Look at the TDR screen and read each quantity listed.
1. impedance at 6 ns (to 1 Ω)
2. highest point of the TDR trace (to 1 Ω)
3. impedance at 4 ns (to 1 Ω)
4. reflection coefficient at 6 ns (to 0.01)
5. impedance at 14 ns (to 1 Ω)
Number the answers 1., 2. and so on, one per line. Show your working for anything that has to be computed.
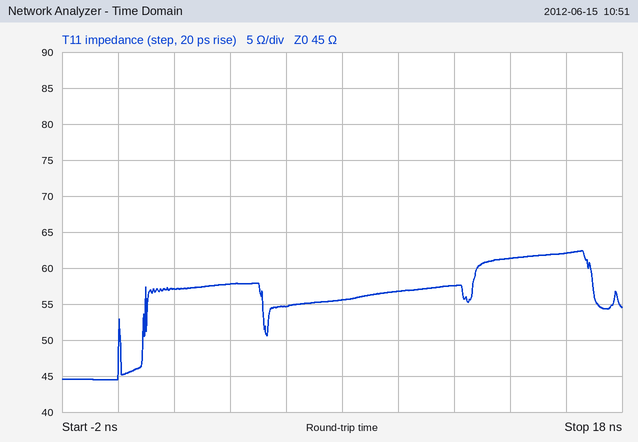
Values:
1. 55 Ω
2. 62 Ω
3. 58 Ω
4. (55 − 45)/(55 + 45) ≈ +0.10
5. 61 Ω
